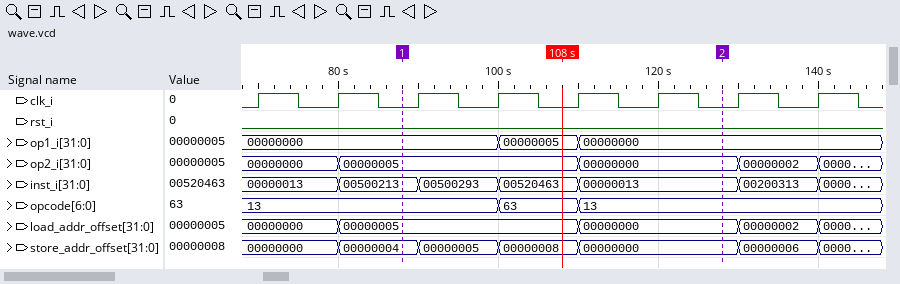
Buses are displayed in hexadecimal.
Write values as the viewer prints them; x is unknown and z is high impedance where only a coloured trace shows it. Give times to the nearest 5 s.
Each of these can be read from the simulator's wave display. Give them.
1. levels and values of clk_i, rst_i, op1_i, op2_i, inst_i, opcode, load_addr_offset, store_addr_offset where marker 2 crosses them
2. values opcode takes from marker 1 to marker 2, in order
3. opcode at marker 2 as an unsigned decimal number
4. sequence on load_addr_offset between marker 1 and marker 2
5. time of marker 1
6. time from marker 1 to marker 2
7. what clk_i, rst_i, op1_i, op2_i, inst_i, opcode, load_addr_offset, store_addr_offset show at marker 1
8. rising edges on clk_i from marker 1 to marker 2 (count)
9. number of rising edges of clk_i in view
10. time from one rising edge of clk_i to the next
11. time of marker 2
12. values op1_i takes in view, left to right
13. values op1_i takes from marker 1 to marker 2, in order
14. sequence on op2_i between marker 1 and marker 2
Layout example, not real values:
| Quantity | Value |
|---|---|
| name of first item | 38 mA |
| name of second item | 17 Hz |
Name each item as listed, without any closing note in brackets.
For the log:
| Quantity | Value |
|---|---|
| levels and values of clk_i, rst_i, op1_i, op2_i, inst_i, opcode, load_addr_offset, store_addr_offset where marker 2 crosses them | clk_i=0, rst_i=0, op1_i=00000000, op2_i=00000000, inst_i=00000013, opcode=13, load_addr_offset=00000000, store_addr_offset=00000000 |
| values opcode takes from marker 1 to marker 2, in order | 13, 63, 13 |
| opcode at marker 2 as an unsigned decimal number | 19 |
| sequence on load_addr_offset between marker 1 and marker 2 | 00000005, 00000000 |
| time of marker 1 | 90 s |
| time from marker 1 to marker 2 | 40 s |
| what clk_i, rst_i, op1_i, op2_i, inst_i, opcode, load_addr_offset, store_addr_offset show at marker 1 | clk_i=0, rst_i=0, op1_i=00000000, op2_i=00000005, inst_i=00500213, opcode=13, load_addr_offset=00000005, store_addr_offset=00000004 |
| rising edges on clk_i from marker 1 to marker 2 | 4 |
| number of rising edges of clk_i in view | 8 |
| time from one rising edge of clk_i to the next | 10 s |
| time of marker 2 | 130 s |
| values op1_i takes in view, left to right | 00000000, 00000005, 00000000 |
| values op1_i takes from marker 1 to marker 2, in order | 00000000, 00000005, 00000000 |
| sequence on op2_i between marker 1 and marker 2 | 00000005, 00000000 |
